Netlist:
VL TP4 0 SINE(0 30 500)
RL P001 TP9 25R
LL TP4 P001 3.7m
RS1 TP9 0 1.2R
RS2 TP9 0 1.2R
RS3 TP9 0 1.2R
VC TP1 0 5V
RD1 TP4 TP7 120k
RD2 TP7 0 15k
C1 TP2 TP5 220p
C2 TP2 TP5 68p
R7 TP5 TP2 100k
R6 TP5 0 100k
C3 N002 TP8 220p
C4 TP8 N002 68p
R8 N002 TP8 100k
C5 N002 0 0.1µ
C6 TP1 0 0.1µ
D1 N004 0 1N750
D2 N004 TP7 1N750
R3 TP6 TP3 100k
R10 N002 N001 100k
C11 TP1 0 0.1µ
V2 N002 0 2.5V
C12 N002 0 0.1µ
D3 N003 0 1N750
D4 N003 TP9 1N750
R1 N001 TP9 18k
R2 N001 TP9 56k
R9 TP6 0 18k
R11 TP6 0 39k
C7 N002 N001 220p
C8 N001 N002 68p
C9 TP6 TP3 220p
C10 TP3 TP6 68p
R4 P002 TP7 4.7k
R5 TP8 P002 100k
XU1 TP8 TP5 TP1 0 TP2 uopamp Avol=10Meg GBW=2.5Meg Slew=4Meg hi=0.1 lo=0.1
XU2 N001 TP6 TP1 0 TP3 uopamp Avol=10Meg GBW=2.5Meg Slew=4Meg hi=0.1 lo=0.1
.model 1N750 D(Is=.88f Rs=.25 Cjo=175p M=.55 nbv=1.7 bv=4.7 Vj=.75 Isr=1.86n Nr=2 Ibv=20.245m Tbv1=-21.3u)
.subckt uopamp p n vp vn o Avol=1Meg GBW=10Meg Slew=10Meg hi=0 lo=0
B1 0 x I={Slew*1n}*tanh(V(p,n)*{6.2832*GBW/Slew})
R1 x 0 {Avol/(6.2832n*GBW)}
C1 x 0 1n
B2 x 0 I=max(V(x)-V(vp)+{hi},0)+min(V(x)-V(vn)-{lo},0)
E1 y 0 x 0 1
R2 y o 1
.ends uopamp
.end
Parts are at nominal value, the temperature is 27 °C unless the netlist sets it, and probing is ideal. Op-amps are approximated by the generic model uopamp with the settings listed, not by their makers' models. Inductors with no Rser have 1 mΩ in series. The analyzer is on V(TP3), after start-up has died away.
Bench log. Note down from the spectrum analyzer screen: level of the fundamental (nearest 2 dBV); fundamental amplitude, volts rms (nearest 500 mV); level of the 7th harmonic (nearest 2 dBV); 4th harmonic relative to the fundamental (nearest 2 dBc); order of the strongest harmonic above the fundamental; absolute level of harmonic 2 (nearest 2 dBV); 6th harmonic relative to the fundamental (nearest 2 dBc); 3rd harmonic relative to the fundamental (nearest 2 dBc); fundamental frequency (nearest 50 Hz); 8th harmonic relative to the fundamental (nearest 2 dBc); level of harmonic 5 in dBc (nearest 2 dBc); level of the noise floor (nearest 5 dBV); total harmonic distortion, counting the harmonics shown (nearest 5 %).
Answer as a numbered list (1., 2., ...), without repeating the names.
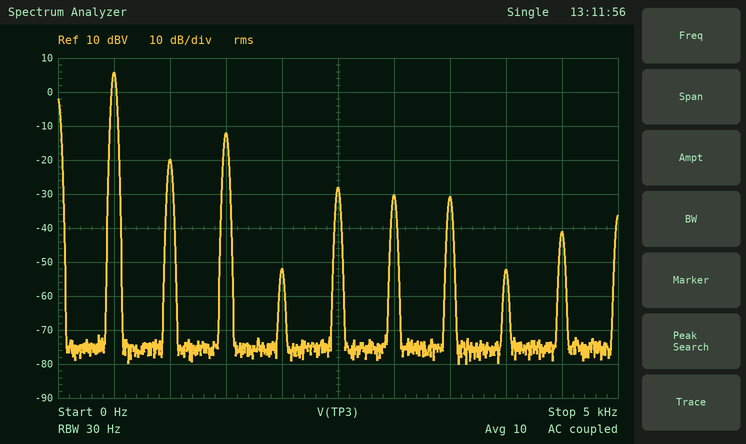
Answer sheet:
1. 6 dBV
2. 2.0 V
3. -30 dBV
4. -58 dBc
5. 3
6. -20 dBV
7. -36 dBc
8. -18 dBc
9. 500 Hz
10. -58 dBc
11. -34 dBc
12. -75 dBV
13. 15 %
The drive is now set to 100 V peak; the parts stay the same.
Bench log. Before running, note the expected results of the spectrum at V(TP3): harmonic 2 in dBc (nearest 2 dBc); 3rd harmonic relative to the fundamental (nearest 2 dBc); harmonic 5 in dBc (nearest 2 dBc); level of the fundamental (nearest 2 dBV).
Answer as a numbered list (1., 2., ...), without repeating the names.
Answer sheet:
1. -34 dBc
2. -10 dBc
3. -16 dBc
4. 6 dBV
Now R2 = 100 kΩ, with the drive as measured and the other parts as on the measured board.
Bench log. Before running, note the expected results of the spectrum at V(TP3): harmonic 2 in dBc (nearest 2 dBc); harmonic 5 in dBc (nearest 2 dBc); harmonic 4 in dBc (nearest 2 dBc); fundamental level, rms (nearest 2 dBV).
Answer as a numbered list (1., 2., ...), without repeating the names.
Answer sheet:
1. -18 dBc
2. -42 dBc
3. -52 dBc
4. 6 dBV
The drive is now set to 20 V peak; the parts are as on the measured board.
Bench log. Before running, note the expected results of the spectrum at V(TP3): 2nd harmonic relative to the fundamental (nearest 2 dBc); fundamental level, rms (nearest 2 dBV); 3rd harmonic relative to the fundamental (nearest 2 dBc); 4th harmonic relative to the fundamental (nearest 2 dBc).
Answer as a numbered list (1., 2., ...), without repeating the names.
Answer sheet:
1. -42 dBc
2. 4 dBV
3. -44 dBc
4. -44 dBc
